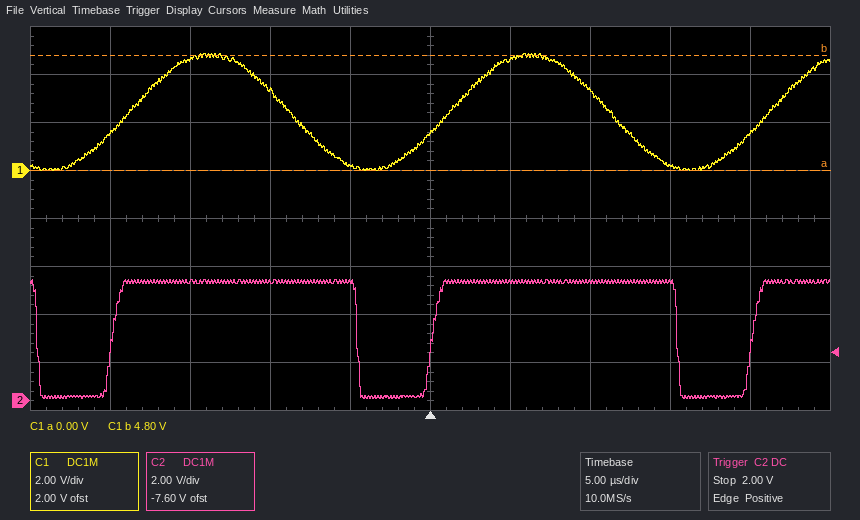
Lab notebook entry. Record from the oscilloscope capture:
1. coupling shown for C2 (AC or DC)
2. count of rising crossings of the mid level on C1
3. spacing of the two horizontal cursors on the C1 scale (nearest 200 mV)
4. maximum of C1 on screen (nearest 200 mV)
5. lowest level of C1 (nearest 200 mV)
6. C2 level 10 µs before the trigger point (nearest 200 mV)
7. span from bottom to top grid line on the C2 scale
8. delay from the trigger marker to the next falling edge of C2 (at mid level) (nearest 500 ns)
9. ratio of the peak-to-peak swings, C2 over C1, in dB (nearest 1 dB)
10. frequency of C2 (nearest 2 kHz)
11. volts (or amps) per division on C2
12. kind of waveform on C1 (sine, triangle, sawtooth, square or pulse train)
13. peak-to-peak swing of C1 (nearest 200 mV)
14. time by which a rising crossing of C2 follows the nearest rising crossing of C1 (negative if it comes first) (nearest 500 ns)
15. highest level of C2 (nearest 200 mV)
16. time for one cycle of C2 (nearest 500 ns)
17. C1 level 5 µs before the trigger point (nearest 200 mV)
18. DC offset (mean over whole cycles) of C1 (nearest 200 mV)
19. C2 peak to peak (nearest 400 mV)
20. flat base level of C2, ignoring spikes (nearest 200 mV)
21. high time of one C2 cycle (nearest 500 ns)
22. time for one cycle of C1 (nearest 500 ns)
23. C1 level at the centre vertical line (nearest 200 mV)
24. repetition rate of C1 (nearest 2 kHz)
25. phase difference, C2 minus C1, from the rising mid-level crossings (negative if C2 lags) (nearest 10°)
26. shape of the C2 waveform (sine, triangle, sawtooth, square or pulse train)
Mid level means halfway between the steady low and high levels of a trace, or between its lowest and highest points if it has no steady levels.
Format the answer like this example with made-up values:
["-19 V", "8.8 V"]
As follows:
["DC", "3", "4.8 V", "4.8 V", "0.0 V", "5.0 V", "16 V", "15.5 µs", "0 dB", "50 kHz", "2 V", "sine", "4.8 V", "-1.0 µs", "5.0 V", "20.0 µs", "200 mV", "2.4 V", "4.8 V", "200 mV", "15.5 µs", "20.0 µs", "1.6 V", "50 kHz", "+20°", "pulse train"]
